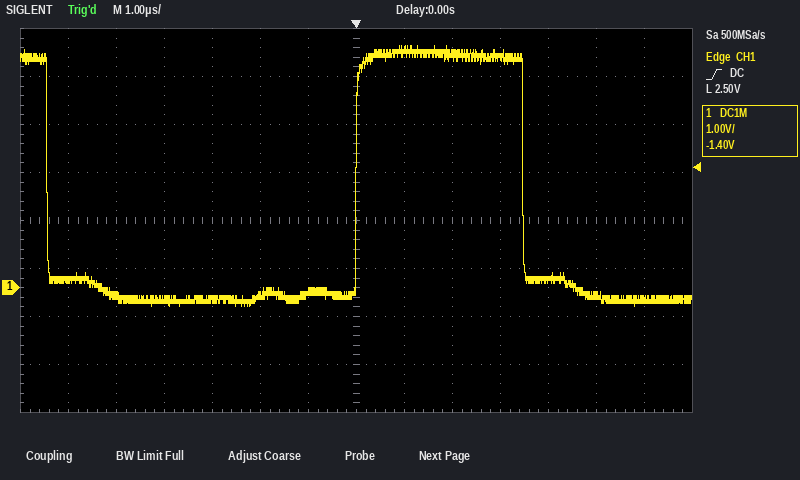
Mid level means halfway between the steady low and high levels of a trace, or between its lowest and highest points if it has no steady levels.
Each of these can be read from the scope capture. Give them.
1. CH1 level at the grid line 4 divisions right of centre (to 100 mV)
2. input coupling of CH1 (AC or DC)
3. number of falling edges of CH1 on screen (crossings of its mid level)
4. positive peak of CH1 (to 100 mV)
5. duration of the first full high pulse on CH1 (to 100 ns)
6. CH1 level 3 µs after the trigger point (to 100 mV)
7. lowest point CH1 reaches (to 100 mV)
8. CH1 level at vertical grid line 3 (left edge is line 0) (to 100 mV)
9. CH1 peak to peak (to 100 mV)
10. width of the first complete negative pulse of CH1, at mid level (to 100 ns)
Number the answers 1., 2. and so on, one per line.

1. 200 mV
2. DC
3. 2
4. 5.0 V
5. 3.5 µs
6. 4.8 V
7. -400 mV
8. -200 mV
9. 5.4 V
10. 6.4 µs
